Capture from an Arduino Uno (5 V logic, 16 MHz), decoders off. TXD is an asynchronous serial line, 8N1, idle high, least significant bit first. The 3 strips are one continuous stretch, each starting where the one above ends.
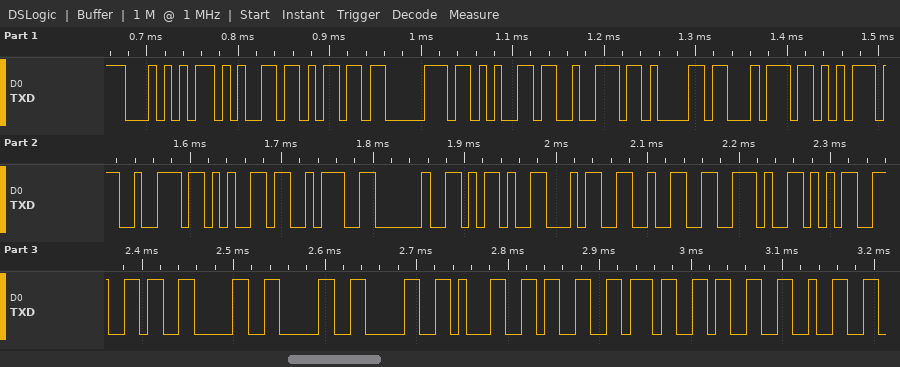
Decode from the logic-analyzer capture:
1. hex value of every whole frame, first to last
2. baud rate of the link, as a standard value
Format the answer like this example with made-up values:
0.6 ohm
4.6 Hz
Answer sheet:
0x54 0x65 0x6D 0x70 0x65 0x72 0x61 0x74 0x75 0x72 0x65 0x3A 0x20 0x2D 0x34 0x32 0x2E 0x35 0x36 0x30 0x30 0x30 0x31 0x33 0x37 0x33 0x32
115200 baud
